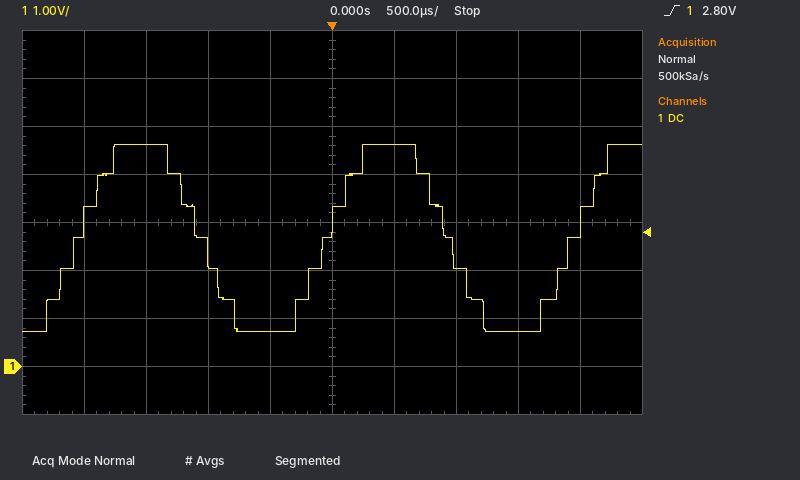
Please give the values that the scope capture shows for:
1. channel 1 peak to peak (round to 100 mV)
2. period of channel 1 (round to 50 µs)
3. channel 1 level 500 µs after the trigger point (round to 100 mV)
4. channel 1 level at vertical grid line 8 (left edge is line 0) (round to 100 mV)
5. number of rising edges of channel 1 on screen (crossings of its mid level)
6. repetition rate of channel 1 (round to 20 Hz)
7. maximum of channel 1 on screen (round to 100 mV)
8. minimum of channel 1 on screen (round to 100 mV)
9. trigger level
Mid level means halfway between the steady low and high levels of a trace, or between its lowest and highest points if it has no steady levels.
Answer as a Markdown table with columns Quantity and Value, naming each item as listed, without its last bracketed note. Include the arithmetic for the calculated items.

| Quantity | Value |
|---|---|
| channel 1 peak to peak | 4.6 V − (700 mV) = 3.9 V |
| period of channel 1 | 2.00 ms |
| channel 1 level 500 µs after the trigger point | 4.6 V |
| channel 1 level at vertical grid line 8 (left edge is line 0) | 700 mV |
| number of rising edges of channel 1 on screen | 3 |
| repetition rate of channel 1 | 1 / 2.00 ms ≈ 500 Hz |
| maximum of channel 1 on screen | 4.6 V |
| minimum of channel 1 on screen | 700 mV |
| trigger level | 2.80 V |
